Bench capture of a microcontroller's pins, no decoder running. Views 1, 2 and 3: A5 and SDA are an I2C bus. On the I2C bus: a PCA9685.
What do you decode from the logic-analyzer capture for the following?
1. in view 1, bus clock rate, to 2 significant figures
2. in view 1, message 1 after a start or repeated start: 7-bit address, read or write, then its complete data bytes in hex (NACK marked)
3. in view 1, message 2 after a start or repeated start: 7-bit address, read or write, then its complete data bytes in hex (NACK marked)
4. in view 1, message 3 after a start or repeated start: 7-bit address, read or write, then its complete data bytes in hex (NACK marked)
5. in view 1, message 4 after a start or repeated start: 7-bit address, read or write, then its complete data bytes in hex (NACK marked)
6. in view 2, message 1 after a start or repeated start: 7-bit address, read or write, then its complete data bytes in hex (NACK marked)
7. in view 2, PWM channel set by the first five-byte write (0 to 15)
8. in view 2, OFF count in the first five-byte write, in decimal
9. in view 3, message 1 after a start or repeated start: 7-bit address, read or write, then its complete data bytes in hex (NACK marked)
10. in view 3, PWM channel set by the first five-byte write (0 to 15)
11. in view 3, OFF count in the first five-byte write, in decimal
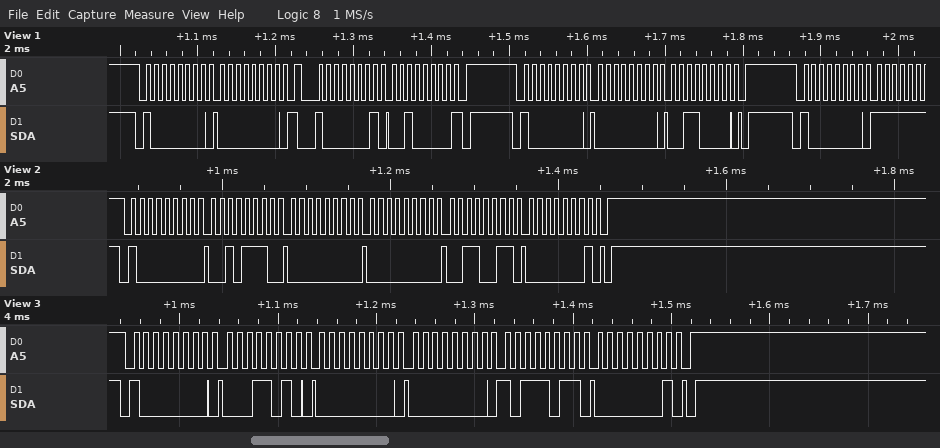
100 kHz
0x40 write: 00
0x40 read: 20 NACK
0x40 write: 00 30
0x40 write
0x40 write: 2E 00 00 33 01
10
307
0x40 write: 1A 00 00 BB 01
5
443
